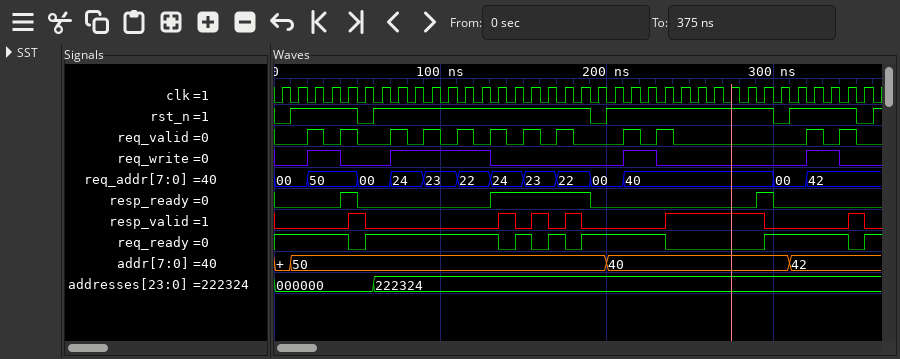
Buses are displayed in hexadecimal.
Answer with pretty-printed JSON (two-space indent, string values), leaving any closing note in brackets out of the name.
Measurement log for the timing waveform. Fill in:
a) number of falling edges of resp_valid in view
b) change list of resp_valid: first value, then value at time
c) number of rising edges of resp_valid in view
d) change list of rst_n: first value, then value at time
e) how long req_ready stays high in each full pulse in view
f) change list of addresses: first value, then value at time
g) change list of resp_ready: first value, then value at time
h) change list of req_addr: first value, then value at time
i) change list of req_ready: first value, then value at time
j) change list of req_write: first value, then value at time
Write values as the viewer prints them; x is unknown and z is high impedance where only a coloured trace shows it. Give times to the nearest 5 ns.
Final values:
{
  "number of falling edges of resp_valid in view": "6",
  "change list of resp_valid: first value, then value at time": "0, 1 at 45 ns, 0 at 55 ns, 1 at 135 ns, 0 at 145 ns, 1 at 155 ns, 0 at 165 ns, 1 at 175 ns, 0 at 185 ns, 1 at 235 ns, 0 at 295 ns, 1 at 345 ns, 0 at 355 ns",
  "number of rising edges of resp_valid in view": "6",
  "change list of rst_n: first value, then value at time": "0, 1 at 10 ns, 0 at 50 ns, 1 at 60 ns, 0 at 190 ns, 1 at 200 ns, 0 at 300 ns, 1 at 310 ns, 0 at 350 ns, 1 at 360 ns",
  "how long req_ready stays high in each full pulse in view": "80 ns, 10 ns, 10 ns, 50 ns, 50 ns",
  "change list of addresses: first value, then value at time": "000000, 222324 at 60 ns",
  "change list of resp_ready: first value, then value at time": "0, 1 at 40 ns, 0 at 50 ns, 1 at 130 ns, 0 at 190 ns, 1 at 290 ns, 0 at 300 ns",
  "change list of req_addr: first value, then value at time": "00, 50 at 20 ns, 00 at 50 ns, 24 at 70 ns, 23 at 90 ns, 22 at 110 ns, 24 at 130 ns, 23 at 150 ns, 22 at 170 ns, 00 at 190 ns, 40 at 210 ns, 00 at 300 ns, 42 at 320 ns",
  "change list of req_ready: first value, then value at time": "1, 0 at 45 ns, 1 at 55 ns, 0 at 135 ns, 1 at 145 ns, 0 at 155 ns, 1 at 165 ns, 0 at 175 ns, 1 at 185 ns, 0 at 235 ns, 1 at 295 ns, 0 at 345 ns, 1 at 355 ns",
  "change list of req_write: first value, then value at time": "0, 1 at 20 ns, 0 at 40 ns, 1 at 70 ns, 0 at 130 ns, 1 at 210 ns, 0 at 230 ns, 1 at 320 ns, 0 at 340 ns"
}
